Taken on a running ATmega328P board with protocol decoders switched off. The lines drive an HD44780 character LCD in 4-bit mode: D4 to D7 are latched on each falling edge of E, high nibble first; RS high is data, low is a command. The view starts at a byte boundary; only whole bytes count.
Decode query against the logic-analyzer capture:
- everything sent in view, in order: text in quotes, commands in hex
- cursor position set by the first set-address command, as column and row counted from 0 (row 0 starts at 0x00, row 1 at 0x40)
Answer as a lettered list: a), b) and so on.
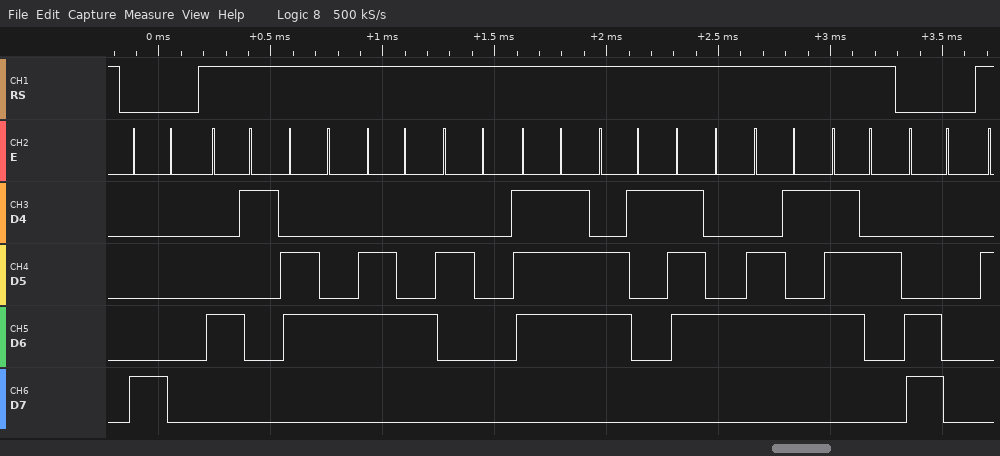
a) 0x80 "Add water" 0xC0
b) column 0, row 0
